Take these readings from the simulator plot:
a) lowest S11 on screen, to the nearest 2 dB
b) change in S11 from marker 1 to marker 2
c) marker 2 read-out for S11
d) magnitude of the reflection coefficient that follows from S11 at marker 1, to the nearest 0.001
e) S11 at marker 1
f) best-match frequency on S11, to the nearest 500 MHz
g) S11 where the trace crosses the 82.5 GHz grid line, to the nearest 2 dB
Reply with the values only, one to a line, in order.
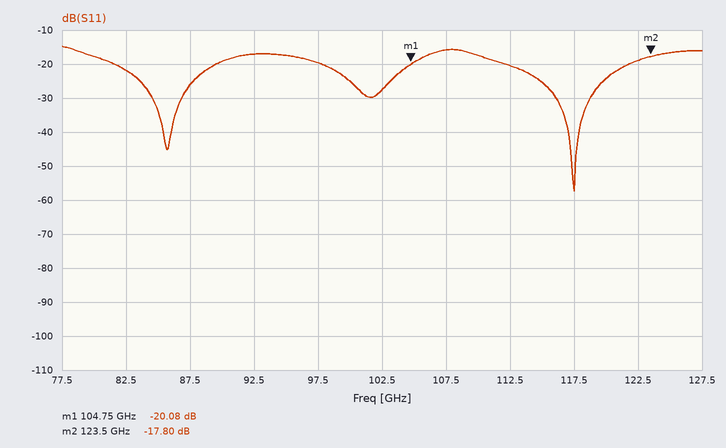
-58 dB
2.28 dB
-17.80 dB
0.099
-20.08 dB
117.5 GHz
-22 dB
